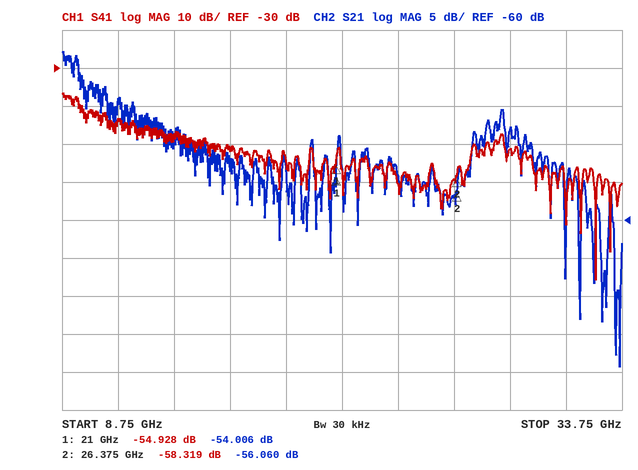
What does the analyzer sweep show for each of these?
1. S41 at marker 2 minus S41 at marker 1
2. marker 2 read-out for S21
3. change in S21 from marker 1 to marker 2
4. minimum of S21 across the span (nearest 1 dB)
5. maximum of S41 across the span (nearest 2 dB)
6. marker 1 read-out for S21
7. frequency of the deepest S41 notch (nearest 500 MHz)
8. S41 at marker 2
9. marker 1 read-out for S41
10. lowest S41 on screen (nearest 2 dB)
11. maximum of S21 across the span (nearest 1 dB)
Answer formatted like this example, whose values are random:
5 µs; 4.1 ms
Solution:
-3.391 dB; -56.060 dB; -2.054 dB; -79 dB; -36 dB; -54.006 dB; 32.5 GHz; -58.319 dB; -54.928 dB; -86 dB; -38 dB
